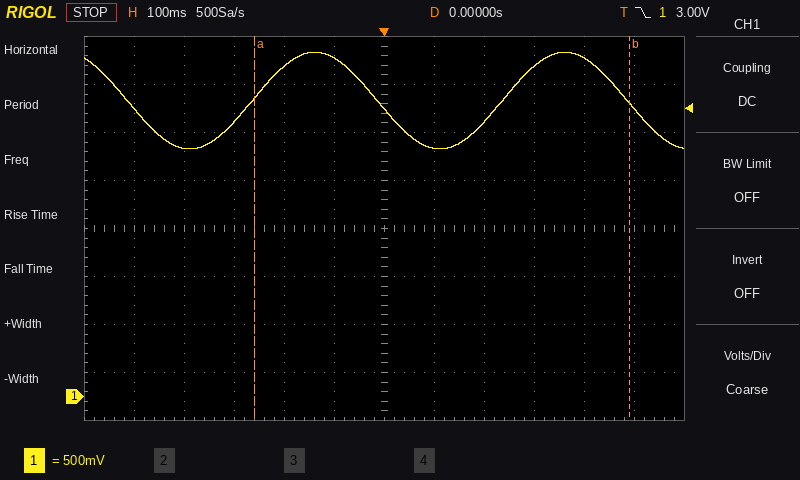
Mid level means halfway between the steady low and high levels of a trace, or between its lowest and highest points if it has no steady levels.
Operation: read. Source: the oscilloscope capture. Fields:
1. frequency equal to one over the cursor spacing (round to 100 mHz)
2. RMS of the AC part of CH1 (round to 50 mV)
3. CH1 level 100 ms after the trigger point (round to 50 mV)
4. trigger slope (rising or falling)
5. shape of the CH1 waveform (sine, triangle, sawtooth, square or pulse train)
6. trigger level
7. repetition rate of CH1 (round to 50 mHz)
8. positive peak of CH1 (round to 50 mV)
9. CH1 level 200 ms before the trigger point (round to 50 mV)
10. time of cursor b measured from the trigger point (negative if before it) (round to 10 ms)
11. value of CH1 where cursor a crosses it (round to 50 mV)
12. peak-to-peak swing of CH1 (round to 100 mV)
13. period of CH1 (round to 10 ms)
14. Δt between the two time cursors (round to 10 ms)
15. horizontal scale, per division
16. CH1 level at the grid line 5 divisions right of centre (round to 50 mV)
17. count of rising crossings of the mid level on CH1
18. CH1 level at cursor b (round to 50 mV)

1.3 Hz
350 mV
2.60 V
falling
sine
3.00 V
2.00 Hz
3.60 V
3.45 V
+490 ms
3.10 V
1.00 V
500 ms
750 ms
100 ms
3.00 V
2
3.05 V
